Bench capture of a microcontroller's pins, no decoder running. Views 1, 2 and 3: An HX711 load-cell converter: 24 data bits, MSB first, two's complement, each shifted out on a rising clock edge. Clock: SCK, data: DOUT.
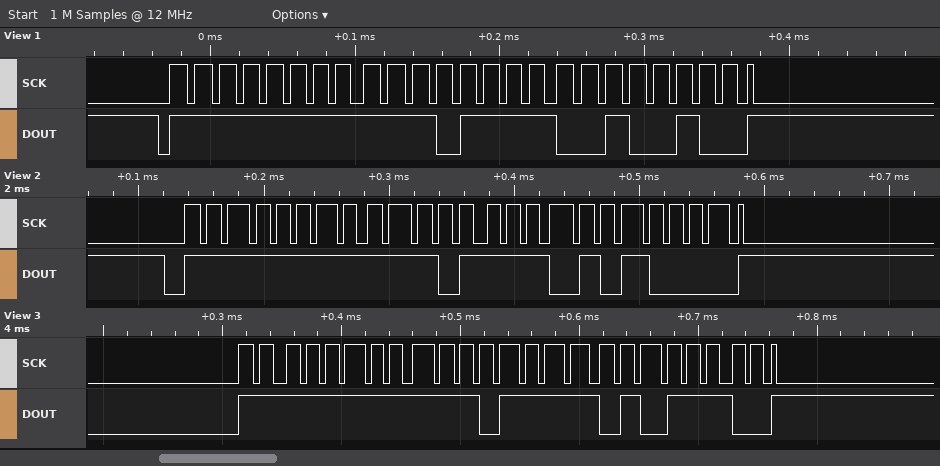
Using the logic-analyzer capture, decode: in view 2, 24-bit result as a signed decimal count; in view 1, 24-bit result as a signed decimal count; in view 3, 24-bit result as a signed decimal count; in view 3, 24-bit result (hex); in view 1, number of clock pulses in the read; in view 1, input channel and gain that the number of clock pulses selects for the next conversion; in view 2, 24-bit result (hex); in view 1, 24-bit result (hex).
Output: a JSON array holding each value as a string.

["-4272", "-4316", "-4260", "0xFFEF5C", "25", "channel A, gain 128", "0xFFEF50", "0xFFEF24"]
